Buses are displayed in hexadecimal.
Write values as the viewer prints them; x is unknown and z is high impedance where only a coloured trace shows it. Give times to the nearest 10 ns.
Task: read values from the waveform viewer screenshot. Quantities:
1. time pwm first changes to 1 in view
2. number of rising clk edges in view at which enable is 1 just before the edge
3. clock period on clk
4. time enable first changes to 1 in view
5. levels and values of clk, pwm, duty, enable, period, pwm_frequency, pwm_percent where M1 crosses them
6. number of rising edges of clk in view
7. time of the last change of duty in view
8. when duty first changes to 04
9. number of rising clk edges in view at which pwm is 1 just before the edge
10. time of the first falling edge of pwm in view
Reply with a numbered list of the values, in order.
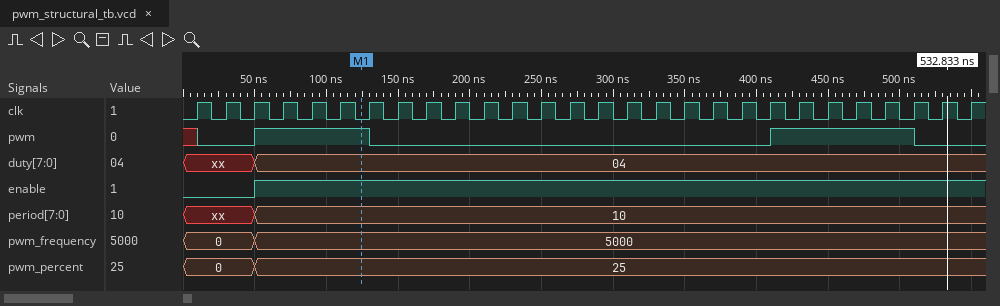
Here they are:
1. 50 ns
2. 25
3. 20 ns
4. 50 ns
5. clk=0, pwm=1, duty=04, enable=1, period=10, pwm_frequency=5000, pwm_percent=25
6. 28
7. 50 ns
8. 50 ns
9. 9
10. 130 ns
